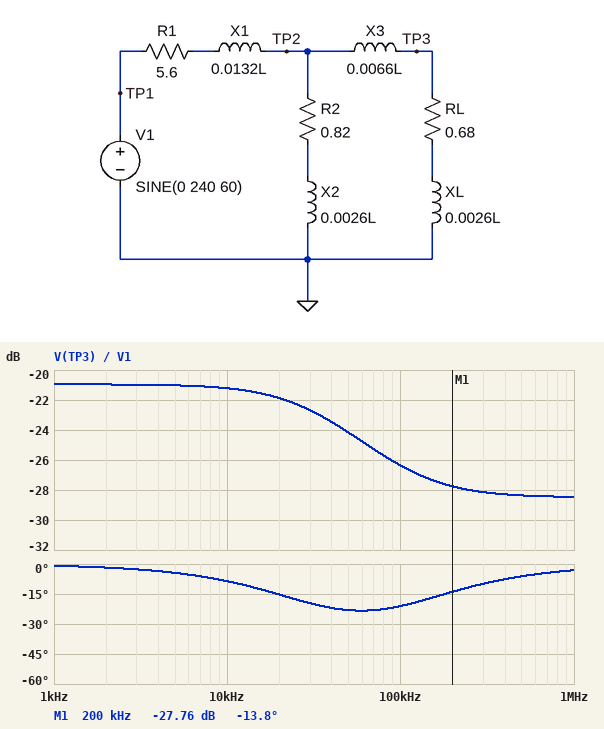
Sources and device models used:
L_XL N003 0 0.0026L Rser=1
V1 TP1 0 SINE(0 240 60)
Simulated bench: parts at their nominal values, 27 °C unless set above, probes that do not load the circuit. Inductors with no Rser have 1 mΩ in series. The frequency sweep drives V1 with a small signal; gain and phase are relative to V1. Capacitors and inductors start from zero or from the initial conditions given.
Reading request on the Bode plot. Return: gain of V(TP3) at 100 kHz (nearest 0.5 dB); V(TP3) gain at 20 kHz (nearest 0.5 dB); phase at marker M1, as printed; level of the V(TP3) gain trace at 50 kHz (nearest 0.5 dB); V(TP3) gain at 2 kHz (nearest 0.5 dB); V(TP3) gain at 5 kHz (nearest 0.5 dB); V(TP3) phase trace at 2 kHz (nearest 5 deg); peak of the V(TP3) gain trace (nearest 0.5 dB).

-26.5 dB
-22.0 dB
-13.8 deg
-24.0 dB
-21.0 dB
-21.0 dB
0 deg
-21.0 dB
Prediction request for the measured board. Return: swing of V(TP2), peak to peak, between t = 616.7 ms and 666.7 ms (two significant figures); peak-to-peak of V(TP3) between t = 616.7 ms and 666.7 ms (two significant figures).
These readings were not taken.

43 V
43 V
